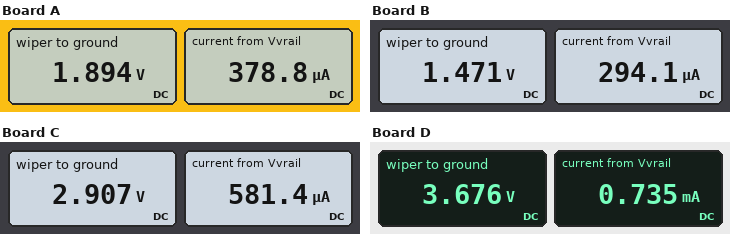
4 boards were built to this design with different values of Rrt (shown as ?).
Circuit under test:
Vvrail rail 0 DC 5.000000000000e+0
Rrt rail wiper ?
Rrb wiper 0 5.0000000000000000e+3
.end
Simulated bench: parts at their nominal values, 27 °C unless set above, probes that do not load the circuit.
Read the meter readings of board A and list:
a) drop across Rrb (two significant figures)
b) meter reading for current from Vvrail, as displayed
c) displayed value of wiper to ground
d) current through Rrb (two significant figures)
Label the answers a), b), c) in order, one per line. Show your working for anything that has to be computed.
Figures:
a) 1.894 V = 1.9 V
b) 378.8 µA
c) 1.894 V
d) (1.894 V) / 5 kΩ = 380 µA
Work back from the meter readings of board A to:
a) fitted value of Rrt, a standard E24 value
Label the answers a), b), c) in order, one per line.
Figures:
a) 8.2 kΩ
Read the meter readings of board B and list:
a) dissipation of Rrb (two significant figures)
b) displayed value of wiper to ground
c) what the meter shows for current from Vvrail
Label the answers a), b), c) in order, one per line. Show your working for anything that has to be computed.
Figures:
a) (1.471 V)^2 / 5 kΩ = 430 µW
b) 1.471 V
c) 294.1 µA
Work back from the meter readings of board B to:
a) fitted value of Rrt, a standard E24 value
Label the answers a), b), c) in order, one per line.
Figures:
a) 12 kΩ
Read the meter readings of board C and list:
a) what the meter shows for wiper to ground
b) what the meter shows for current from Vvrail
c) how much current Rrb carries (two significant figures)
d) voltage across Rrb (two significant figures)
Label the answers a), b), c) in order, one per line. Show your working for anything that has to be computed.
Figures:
a) 2.907 V
b) 581.4 µA
c) (2.907 V) / 5 kΩ = 580 µA
d) 2.907 V = 2.9 V
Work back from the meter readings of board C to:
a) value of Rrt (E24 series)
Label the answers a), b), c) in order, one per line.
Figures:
a) 3.6 kΩ
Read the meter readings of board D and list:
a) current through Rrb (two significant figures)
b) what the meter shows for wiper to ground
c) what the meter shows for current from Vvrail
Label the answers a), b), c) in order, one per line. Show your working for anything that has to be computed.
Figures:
a) (3.676 V) / 5 kΩ = 740 µA
b) 3.676 V
c) 0.735 mA
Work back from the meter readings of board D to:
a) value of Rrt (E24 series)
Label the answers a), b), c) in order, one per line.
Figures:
a) 1.8 kΩ
